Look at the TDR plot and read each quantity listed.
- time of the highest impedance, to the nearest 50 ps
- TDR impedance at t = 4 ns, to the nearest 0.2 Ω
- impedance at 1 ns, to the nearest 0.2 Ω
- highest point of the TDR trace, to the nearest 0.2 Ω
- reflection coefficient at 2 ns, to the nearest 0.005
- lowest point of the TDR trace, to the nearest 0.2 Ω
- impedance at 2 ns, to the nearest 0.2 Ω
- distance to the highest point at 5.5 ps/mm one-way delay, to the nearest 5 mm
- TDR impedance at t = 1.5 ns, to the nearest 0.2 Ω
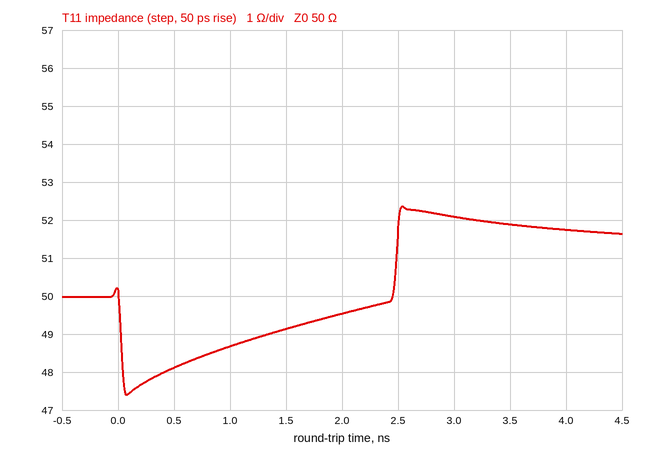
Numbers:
2.55 ns
51.8 Ω
48.6 Ω
52.4 Ω
-0.005
47.4 Ω
49.6 Ω
230 mm
49.2 Ω
